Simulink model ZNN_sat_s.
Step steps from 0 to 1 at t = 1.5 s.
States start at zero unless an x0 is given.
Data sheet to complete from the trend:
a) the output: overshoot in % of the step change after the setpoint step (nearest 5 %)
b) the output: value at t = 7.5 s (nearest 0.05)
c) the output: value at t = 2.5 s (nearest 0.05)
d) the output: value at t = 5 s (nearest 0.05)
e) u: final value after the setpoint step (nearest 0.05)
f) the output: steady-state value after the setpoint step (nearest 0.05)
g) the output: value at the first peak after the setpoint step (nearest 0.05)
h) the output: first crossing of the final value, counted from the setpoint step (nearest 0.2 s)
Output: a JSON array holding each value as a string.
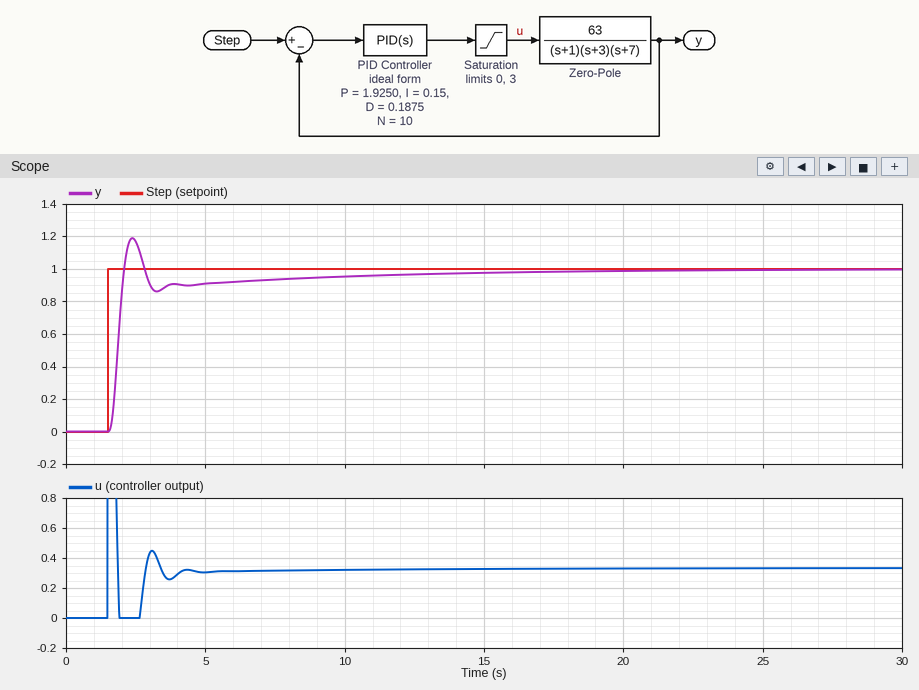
["20 %", "0.95", "1.15", "0.90", "0.35", "1.00", "1.20", "0.6 s"]
